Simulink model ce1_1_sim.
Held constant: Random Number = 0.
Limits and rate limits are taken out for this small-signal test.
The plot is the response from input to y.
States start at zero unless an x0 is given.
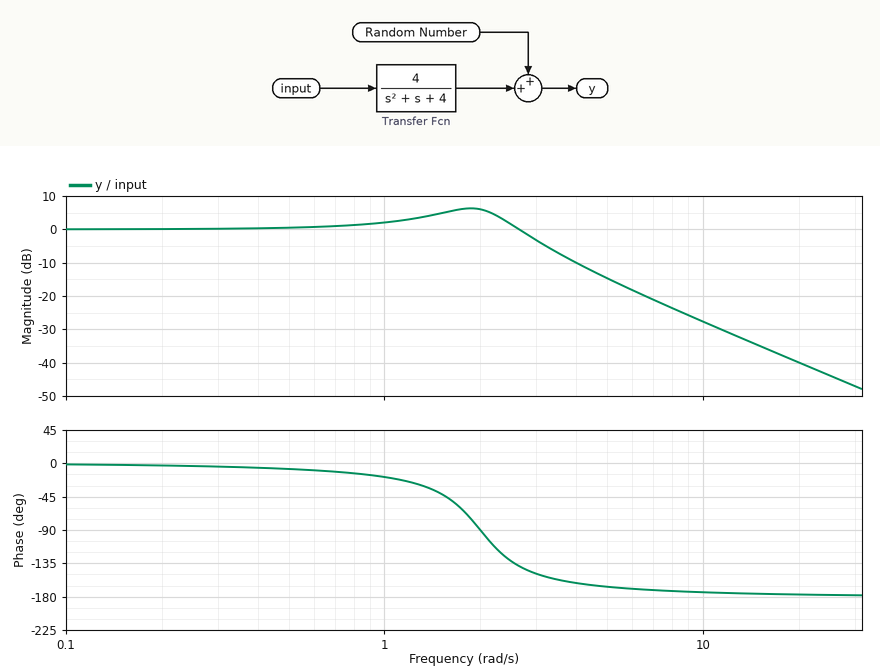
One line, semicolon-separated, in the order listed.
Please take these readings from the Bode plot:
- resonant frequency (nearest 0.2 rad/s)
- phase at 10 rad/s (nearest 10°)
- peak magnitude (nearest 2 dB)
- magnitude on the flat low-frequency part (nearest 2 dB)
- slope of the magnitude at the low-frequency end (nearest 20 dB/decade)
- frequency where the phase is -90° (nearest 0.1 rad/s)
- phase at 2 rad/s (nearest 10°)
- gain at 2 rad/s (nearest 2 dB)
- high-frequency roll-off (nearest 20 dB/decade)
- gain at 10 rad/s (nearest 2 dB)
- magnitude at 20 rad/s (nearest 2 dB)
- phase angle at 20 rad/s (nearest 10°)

1.8 rad/s; -170°; 6 dB; 0 dB; 0 dB/decade; 2.0 rad/s; -90°; 6 dB; -40 dB/decade; -28 dB; -40 dB; -180°
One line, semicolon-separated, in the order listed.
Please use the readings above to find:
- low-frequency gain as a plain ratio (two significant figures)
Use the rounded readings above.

1.0
